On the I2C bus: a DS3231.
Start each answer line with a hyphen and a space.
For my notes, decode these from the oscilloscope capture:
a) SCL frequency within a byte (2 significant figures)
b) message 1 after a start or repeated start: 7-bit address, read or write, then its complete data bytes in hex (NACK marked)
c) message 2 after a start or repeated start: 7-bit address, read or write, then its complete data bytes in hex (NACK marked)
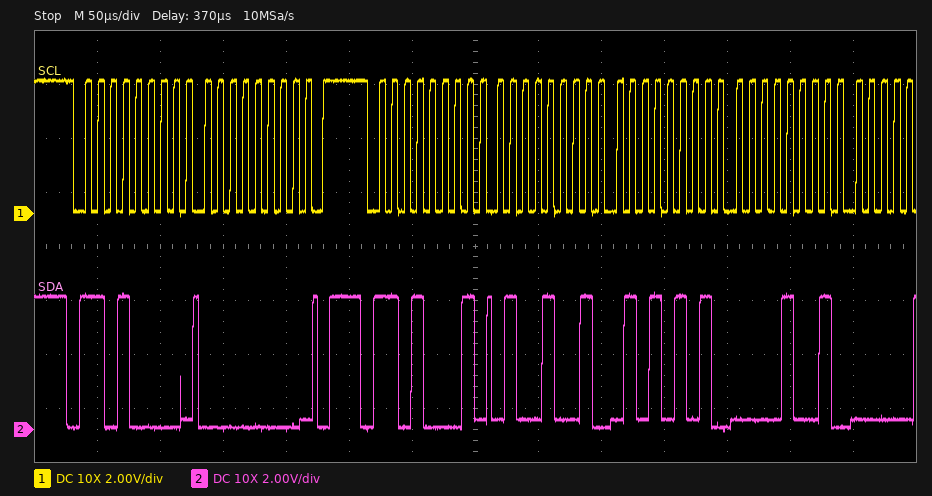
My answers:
- 100 kHz
- 0x68 write: 00
- 0x68 read: 49 55 09
